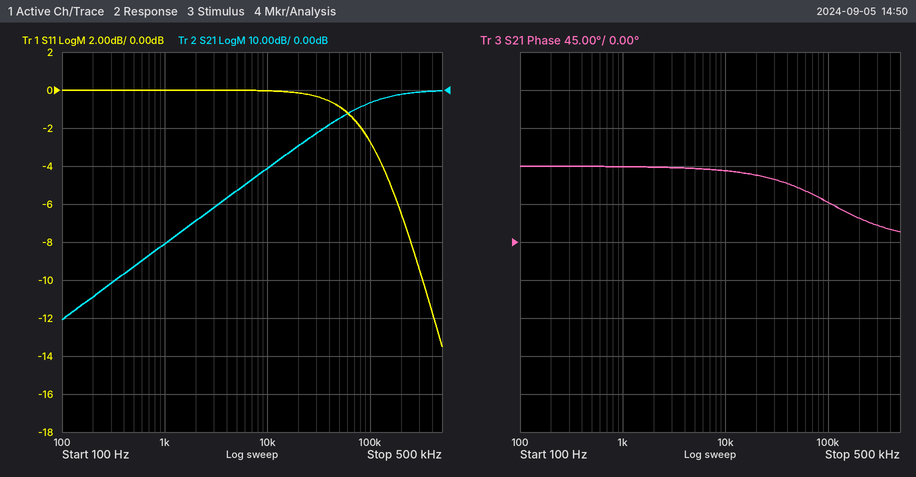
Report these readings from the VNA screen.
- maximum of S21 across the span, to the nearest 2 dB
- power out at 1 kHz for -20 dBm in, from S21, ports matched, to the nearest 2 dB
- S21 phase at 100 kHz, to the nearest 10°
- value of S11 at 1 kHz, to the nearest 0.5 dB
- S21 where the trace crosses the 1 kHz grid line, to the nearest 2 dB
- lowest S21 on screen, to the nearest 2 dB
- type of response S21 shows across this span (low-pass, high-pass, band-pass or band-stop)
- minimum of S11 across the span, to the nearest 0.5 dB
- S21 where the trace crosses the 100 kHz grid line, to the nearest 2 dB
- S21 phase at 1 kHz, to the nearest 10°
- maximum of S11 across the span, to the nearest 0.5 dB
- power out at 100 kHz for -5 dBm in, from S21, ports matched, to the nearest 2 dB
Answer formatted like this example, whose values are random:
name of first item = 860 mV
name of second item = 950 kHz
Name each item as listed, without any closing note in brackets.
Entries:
maximum of S21 across the span, to the nearest 2 dB = 0 dB
power out at 1 kHz for -20 dBm in, from S21, ports matched, to the nearest 2 dB = -60 dBm
S21 phase at 100 kHz, to the nearest 10° = 50°
value of S11 at 1 kHz, to the nearest 0.5 dB = 0.0 dB
S21 where the trace crosses the 1 kHz grid line, to the nearest 2 dB = -40 dB
lowest S21 on screen, to the nearest 2 dB = -60 dB
type of response S21 shows across this span = high-pass
minimum of S11 across the span, to the nearest 0.5 dB = -13.5 dB
S21 where the trace crosses the 100 kHz grid line, to the nearest 2 dB = -4 dB
S21 phase at 1 kHz, to the nearest 10° = 90°
maximum of S11 across the span, to the nearest 0.5 dB = 0.0 dB
power out at 100 kHz for -5 dBm in, from S21, ports matched, to the nearest 2 dB = -8 dBm
